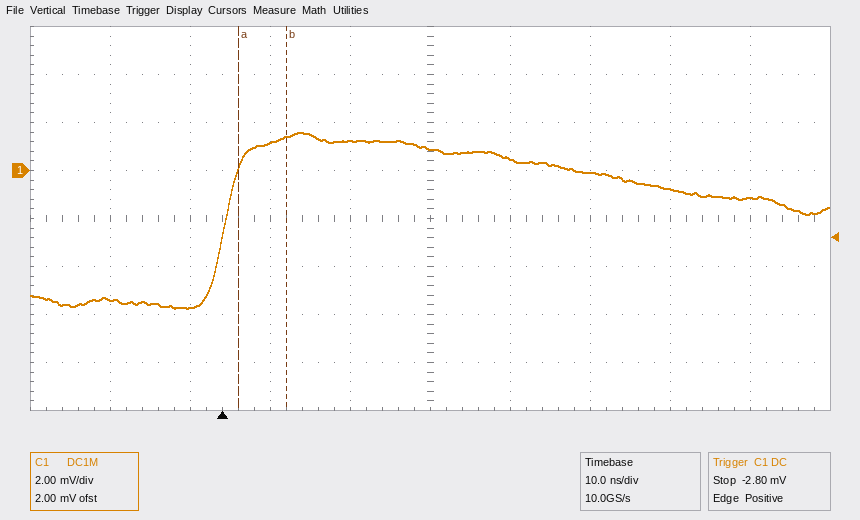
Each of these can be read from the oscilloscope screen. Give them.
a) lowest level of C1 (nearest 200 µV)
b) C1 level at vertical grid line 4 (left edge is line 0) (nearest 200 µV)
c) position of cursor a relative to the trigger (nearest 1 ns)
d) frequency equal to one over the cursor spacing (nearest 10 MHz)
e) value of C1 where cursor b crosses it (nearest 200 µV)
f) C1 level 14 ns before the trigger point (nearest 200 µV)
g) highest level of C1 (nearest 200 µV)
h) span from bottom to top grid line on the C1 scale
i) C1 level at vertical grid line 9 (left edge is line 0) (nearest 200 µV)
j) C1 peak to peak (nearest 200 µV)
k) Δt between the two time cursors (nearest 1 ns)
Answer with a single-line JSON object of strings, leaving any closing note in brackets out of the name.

{"lowest level of C1": "-5.8 mV", "C1 level at vertical grid line 4 (left edge is line 0)": "1.2 mV", "position of cursor a relative to the trigger": "+2 ns", "frequency equal to one over the cursor spacing": "170 MHz", "value of C1 where cursor b crosses it": "1.4 mV", "C1 level 14 ns before the trigger point": "-5.4 mV", "highest level of C1": "1.6 mV", "span from bottom to top grid line on the C1 scale": "16 mV", "C1 level at vertical grid line 9 (left edge is line 0)": "-1.2 mV", "C1 peak to peak": "7.4 mV", "Δt between the two time cursors": "6 ns"}
